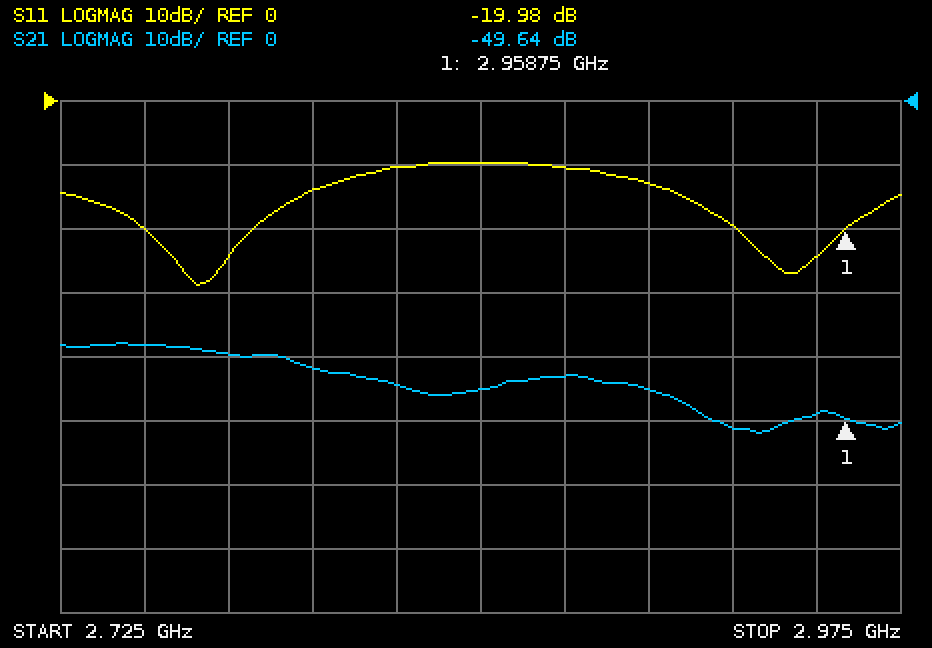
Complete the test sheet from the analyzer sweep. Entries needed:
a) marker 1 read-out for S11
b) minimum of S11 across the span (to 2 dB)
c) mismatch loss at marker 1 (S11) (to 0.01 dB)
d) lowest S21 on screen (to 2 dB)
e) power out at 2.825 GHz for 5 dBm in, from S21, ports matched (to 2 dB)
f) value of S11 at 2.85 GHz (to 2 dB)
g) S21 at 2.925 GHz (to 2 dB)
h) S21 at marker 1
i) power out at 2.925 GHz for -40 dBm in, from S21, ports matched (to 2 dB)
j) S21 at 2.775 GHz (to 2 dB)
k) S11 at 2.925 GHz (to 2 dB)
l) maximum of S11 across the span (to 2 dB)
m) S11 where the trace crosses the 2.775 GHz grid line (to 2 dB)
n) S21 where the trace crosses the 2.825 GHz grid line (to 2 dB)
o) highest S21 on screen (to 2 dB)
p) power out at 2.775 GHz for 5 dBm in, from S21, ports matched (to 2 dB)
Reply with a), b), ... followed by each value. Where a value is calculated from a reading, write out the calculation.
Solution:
a) -19.98 dB
b) -28 dB
c) −10 log10(1 − 10^(-19.98/10)) ≈ 0.04 dB
d) -52 dB
e) 5 dBm + (-44 dB) = -40 dBm
f) -10 dB
g) -52 dB
h) -49.64 dB
i) -40 dBm + (-52 dB) = -92 dBm
j) -40 dB
k) -20 dB
l) -10 dB
m) -24 dB
n) -44 dB
o) -38 dB
p) 5 dBm + (-40 dB) = -34 dBm
